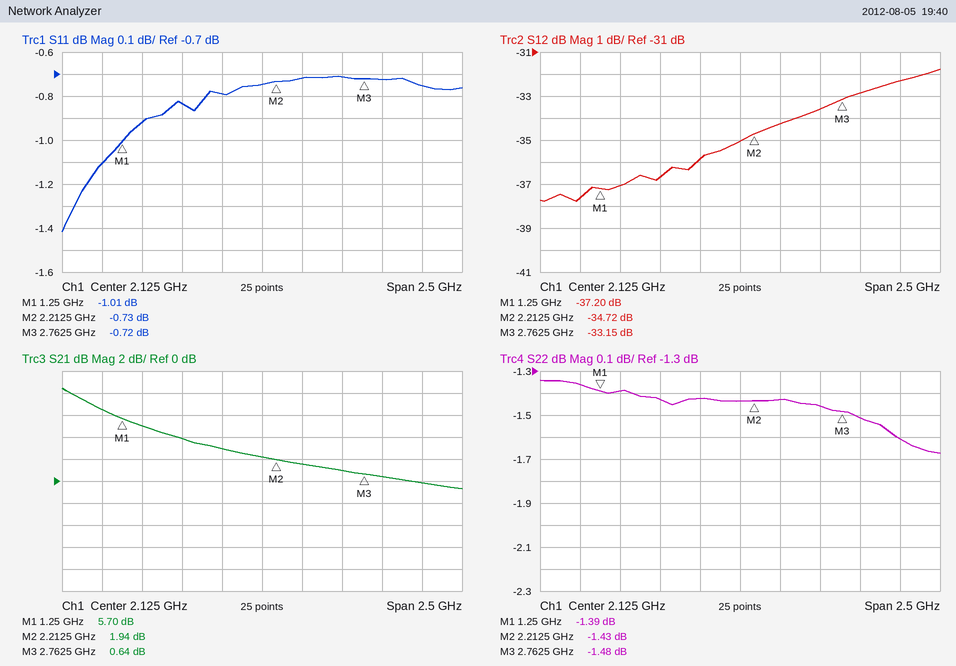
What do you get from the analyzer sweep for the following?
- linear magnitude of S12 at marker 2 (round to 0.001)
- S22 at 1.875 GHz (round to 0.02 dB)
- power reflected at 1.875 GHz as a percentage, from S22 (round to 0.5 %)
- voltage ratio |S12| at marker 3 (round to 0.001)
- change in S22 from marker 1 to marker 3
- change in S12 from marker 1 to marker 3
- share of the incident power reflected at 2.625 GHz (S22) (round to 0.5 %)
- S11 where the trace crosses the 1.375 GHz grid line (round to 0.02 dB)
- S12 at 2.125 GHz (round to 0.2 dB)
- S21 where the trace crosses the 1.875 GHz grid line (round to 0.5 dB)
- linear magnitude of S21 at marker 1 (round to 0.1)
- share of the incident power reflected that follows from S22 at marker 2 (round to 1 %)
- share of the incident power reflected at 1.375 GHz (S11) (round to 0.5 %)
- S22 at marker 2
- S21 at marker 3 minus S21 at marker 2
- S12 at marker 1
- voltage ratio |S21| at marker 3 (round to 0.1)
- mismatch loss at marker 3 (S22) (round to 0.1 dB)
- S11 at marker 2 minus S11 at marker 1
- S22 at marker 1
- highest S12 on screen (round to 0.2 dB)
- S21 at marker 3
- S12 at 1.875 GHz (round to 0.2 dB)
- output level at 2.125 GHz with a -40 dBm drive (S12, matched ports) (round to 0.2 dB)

0.018
-1.42 dB
72.0 %
0.022
-0.09 dB
4.05 dB
71.5 %
-0.92 dB
-35.0 dB
3.0 dB
1.9
72 %
81.0 %
-1.43 dB
-1.30 dB
-37.20 dB
1.1
5.4 dB
0.28 dB
-1.39 dB
-31.8 dB
0.64 dB
-35.8 dB
-75.0 dBm
